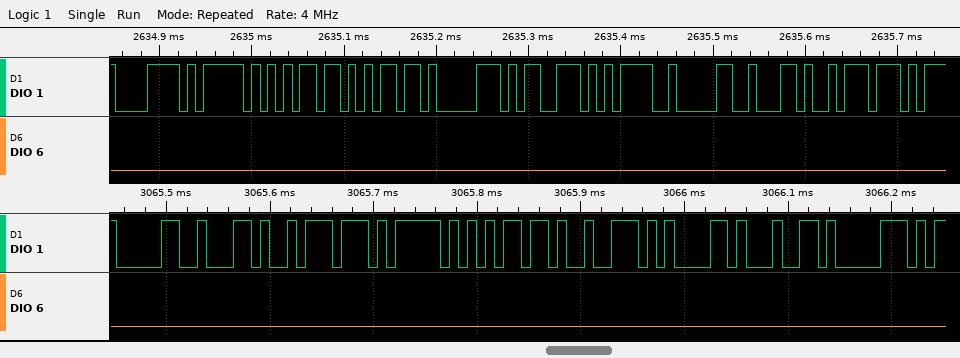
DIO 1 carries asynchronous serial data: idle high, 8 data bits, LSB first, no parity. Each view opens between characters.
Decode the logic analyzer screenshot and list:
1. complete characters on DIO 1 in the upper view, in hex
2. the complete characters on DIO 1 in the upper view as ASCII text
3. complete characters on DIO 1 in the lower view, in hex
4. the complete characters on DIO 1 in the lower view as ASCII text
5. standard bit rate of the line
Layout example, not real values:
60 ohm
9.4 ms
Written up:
78, 5F, 6D, 6D, 70, 73, 3D, 30, 2C, 77
"x_mmps=0,w"
30, 2C, 77, 5F, 6D, 72, 61, 64, 70
"0,w_mradp"
115200 baud
